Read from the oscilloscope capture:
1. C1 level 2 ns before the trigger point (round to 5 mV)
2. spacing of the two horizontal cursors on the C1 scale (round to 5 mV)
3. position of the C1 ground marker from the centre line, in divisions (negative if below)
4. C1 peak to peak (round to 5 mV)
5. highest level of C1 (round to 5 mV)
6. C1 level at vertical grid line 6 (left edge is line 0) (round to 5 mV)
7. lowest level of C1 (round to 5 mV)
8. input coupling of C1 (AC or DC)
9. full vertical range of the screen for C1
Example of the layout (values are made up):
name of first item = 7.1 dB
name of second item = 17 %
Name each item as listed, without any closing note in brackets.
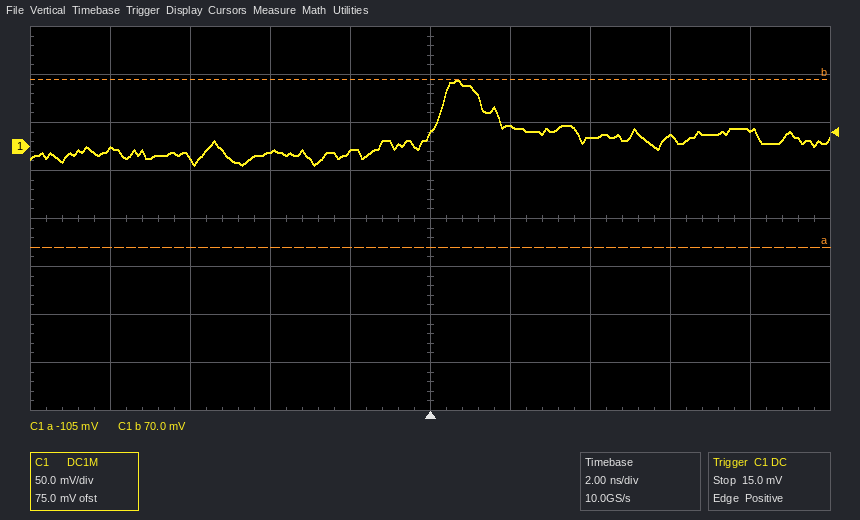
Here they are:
C1 level 2 ns before the trigger point = -5 mV
spacing of the two horizontal cursors on the C1 scale = 175 mV
position of the C1 ground marker from the centre line, in divisions = +1.5 div
C1 peak to peak = 90 mV
highest level of C1 = 70 mV
C1 level at vertical grid line 6 (left edge is line 0) = 20 mV
lowest level of C1 = -20 mV
input coupling of C1 = DC
full vertical range of the screen for C1 = 400 mV
